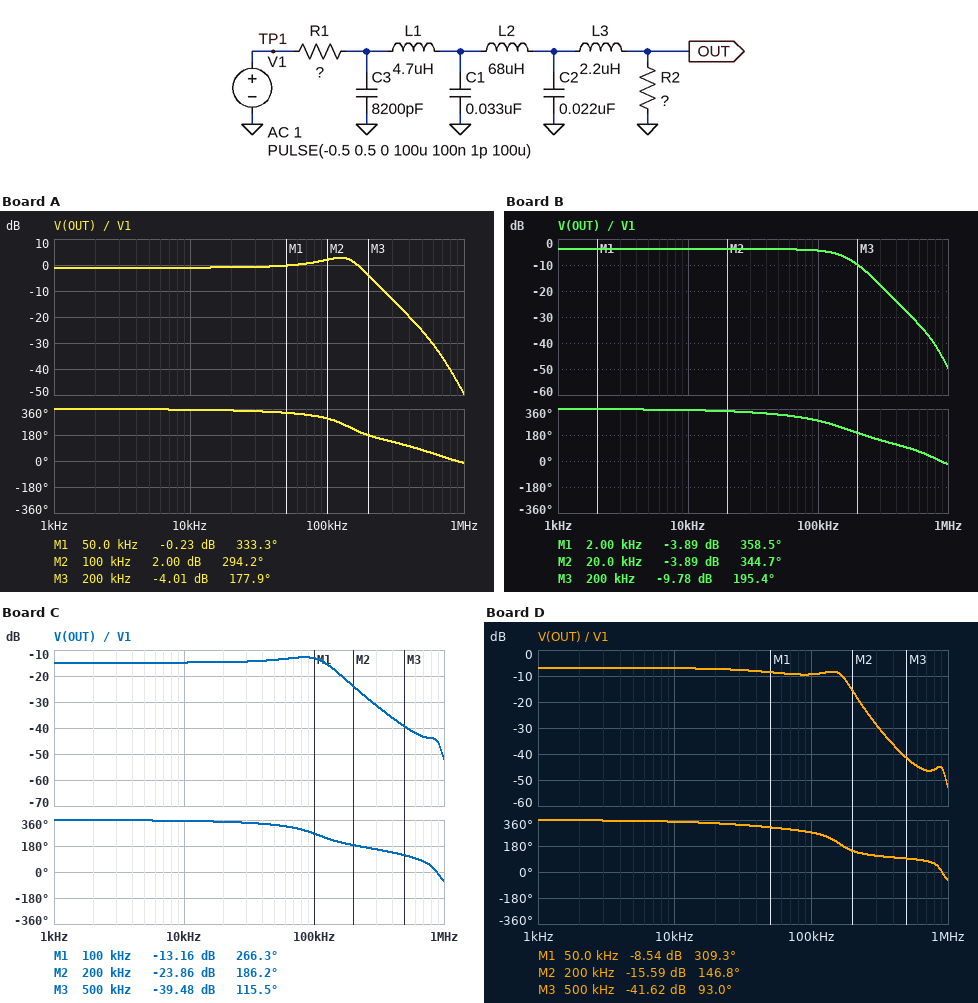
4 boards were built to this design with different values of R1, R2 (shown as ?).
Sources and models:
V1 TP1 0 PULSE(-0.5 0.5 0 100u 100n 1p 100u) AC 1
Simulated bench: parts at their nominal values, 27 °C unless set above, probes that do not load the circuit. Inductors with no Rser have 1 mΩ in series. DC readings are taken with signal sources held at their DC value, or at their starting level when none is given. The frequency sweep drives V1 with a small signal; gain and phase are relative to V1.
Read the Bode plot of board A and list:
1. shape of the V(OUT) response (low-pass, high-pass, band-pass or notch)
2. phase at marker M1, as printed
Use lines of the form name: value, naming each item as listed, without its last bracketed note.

shape of the V(OUT) response: low-pass
phase at marker M1, as printed: 333.3 deg
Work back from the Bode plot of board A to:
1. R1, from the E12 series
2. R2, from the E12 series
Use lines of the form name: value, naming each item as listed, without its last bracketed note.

R1, from the E12 series: 15 Ω
R2, from the E12 series: 120 Ω
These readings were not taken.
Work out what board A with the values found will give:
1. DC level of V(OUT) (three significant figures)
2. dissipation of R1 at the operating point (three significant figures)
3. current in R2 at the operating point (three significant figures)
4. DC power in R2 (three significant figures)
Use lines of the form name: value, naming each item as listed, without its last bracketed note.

DC level of V(OUT): -444 mV
dissipation of R1 at the operating point: 206 µW
current in R2 at the operating point: 3.70 mA
DC power in R2: 1.65 mW
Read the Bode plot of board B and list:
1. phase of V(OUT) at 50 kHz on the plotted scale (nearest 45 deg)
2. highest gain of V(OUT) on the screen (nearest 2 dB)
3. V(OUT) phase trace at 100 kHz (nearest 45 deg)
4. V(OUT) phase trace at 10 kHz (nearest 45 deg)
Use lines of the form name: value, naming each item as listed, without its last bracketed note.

phase of V(OUT) at 50 kHz on the plotted scale: 315 deg
highest gain of V(OUT) on the screen: -4 dB
V(OUT) phase trace at 100 kHz: 270 deg
V(OUT) phase trace at 10 kHz: 360 deg
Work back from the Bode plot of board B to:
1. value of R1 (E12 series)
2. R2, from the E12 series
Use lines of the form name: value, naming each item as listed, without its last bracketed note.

value of R1: 22 Ω
R2, from the E12 series: 39 Ω
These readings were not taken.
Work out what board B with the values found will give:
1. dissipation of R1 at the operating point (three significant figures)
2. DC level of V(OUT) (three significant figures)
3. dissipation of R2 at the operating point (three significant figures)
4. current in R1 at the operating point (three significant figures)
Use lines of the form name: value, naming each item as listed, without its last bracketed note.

dissipation of R1 at the operating point: 1.48 mW
DC level of V(OUT): -320 mV
dissipation of R2 at the operating point: 2.62 mW
current in R1 at the operating point: 8.20 mA
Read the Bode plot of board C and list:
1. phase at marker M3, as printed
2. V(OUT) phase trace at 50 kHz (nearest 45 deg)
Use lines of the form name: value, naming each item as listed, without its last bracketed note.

phase at marker M3, as printed: 115.5 deg
V(OUT) phase trace at 50 kHz: 315 deg
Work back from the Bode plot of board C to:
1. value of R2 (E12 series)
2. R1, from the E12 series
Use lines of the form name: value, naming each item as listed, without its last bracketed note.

value of R2: 15 Ω
R1, from the E12 series: 68 Ω
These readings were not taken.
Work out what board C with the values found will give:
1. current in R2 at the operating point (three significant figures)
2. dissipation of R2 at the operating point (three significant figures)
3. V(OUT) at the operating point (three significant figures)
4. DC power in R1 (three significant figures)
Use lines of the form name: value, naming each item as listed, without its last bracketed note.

current in R2 at the operating point: 6.02 mA
dissipation of R2 at the operating point: 544 µW
V(OUT) at the operating point: -90.4 mV
DC power in R1: 2.47 mW
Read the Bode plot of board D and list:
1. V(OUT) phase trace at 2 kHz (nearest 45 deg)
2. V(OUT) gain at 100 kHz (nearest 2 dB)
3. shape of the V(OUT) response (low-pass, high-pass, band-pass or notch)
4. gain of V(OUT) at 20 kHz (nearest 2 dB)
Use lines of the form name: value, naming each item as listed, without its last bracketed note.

V(OUT) phase trace at 2 kHz: 360 deg
V(OUT) gain at 100 kHz: -10 dB
shape of the V(OUT) response: low-pass
gain of V(OUT) at 20 kHz: -8 dB
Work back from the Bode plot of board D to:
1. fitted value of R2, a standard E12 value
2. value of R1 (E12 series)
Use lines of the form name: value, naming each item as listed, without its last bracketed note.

fitted value of R2, a standard E12 value: 82 Ω
value of R1: 100 Ω
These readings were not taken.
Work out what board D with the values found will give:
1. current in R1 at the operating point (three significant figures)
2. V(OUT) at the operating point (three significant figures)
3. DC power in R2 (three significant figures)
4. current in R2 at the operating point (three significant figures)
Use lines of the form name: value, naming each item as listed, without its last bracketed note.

current in R1 at the operating point: 2.75 mA
V(OUT) at the operating point: -225 mV
DC power in R2: 619 µW
current in R2 at the operating point: 2.75 mA
